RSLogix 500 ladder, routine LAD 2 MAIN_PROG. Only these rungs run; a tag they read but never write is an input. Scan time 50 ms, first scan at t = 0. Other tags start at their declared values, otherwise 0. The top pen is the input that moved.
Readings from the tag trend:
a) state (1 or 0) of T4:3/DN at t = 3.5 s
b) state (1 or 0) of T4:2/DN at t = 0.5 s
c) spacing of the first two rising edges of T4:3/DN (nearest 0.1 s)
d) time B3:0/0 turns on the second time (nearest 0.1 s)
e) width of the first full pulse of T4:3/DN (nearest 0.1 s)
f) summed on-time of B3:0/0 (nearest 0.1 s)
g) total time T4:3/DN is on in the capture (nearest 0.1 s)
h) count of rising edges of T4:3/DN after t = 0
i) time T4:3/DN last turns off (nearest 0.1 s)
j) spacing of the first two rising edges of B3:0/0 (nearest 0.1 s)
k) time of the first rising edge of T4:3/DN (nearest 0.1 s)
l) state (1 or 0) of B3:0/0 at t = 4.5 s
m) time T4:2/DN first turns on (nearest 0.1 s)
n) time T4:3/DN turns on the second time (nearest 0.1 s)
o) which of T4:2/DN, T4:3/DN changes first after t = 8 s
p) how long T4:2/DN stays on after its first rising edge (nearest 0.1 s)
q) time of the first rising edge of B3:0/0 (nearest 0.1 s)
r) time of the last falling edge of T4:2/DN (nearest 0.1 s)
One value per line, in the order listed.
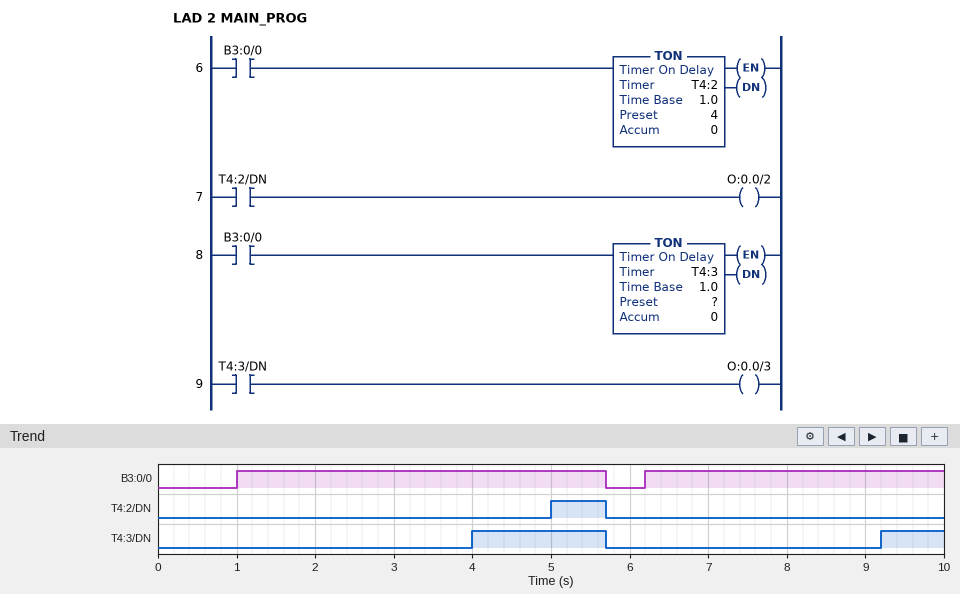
0
0
5.2 s
6.2 s
1.7 s
8.5 s
2.5 s
2
5.7 s
5.2 s
4.0 s
1
5.0 s
9.2 s
T4:3/DN
0.7 s
1.0 s
5.7 s
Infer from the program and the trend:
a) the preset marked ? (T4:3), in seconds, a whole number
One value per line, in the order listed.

3 s
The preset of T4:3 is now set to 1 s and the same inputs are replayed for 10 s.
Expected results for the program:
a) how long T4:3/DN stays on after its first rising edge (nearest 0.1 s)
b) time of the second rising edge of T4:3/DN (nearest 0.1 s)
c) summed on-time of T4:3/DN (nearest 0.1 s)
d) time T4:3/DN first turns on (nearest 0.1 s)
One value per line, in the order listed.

3.7 s
7.2 s
6.5 s
2.0 s
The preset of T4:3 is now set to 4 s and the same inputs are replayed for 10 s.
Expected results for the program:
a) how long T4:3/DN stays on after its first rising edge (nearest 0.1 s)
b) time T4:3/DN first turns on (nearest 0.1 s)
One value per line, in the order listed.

0.7 s
5.0 s
